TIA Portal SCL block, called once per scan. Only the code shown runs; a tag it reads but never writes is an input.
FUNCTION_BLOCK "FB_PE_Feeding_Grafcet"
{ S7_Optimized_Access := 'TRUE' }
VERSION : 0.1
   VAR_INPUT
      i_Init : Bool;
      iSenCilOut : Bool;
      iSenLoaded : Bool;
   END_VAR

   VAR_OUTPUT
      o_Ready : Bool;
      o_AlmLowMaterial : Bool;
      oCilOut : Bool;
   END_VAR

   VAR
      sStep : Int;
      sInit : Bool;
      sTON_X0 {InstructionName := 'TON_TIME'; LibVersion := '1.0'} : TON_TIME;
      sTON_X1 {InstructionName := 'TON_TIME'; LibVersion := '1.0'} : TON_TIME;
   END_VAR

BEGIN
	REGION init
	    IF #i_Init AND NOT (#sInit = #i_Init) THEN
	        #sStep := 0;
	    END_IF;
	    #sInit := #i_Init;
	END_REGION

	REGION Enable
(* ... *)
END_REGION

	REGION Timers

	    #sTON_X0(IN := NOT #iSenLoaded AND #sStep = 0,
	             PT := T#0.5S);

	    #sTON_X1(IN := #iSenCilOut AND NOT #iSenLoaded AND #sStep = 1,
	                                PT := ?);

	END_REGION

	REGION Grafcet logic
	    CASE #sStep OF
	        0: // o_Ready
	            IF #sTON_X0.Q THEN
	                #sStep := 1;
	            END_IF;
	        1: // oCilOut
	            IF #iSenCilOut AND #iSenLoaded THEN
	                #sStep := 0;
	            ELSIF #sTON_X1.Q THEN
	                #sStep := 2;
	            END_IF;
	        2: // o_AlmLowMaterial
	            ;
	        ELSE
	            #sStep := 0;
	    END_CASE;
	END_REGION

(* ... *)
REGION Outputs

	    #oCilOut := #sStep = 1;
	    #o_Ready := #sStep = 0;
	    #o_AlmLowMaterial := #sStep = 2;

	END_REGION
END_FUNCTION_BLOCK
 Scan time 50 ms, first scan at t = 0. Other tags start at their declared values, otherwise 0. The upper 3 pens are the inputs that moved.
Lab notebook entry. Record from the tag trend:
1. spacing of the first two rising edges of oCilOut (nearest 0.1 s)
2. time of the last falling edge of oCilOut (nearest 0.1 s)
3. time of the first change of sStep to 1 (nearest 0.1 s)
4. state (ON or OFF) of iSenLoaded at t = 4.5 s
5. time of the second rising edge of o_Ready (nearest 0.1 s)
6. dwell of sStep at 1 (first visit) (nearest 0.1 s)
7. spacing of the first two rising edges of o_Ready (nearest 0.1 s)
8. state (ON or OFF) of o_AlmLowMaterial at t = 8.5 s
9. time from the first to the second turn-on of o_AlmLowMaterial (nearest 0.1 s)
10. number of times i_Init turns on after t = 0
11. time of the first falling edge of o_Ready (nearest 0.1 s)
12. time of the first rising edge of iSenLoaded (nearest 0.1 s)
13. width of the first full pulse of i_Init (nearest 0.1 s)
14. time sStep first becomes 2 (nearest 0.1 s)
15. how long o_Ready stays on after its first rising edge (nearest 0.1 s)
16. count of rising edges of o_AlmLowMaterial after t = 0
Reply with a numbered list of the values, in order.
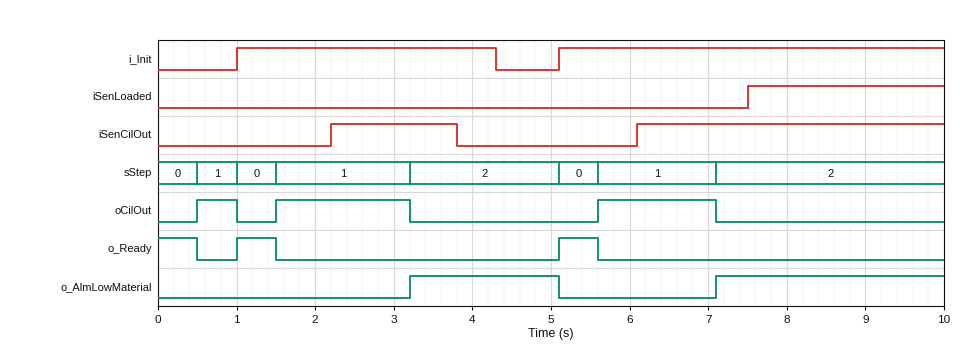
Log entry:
1. 1.0 s
2. 7.1 s
3. 0.5 s
4. OFF
5. 5.1 s
6. 0.5 s
7. 4.1 s
8. ON
9. 3.9 s
10. 2
11. 0.5 s
12. 7.5 s
13. 3.3 s
14. 3.2 s
15. 0.5 s
16. 2
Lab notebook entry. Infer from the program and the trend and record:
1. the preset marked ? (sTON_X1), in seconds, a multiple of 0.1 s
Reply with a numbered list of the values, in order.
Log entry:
1. 1.0 s
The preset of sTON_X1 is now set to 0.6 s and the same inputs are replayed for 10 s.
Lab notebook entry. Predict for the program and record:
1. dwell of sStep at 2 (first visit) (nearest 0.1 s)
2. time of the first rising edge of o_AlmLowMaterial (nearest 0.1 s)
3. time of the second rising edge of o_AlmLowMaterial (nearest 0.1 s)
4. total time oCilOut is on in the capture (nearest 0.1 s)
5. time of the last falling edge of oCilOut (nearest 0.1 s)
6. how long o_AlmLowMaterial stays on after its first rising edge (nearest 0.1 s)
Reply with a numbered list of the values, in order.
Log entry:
1. 2.3 s
2. 2.8 s
3. 6.7 s
4. 2.9 s
5. 6.7 s
6. 2.3 s
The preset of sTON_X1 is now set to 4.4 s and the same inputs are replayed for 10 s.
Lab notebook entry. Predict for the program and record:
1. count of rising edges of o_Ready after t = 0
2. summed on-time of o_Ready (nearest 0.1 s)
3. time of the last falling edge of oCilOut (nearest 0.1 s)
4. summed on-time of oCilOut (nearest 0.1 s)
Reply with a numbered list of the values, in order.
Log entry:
1. 3
2. 4.0 s
3. 7.5 s
4. 6.0 s
